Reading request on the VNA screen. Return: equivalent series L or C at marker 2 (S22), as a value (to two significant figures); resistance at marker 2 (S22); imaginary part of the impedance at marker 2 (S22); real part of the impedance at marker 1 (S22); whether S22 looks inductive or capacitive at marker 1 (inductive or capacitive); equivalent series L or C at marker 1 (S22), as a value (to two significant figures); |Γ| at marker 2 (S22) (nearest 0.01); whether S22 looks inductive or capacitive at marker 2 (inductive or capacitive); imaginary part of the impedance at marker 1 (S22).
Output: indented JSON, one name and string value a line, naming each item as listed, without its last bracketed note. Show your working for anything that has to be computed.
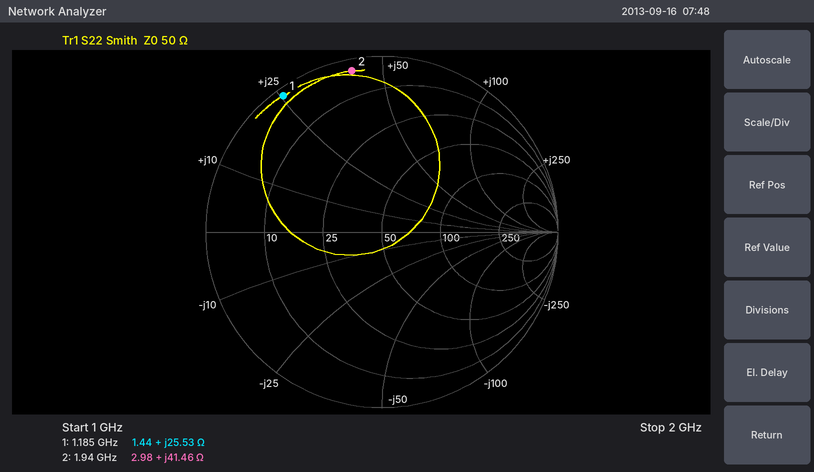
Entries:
{
  "equivalent series L or C at marker 2 (S22), as a value": "L = 41.46 Ω/(2π × 1.94 GHz) ≈ 3.4 nH",
  "resistance at marker 2": "2.98 Ω",
  "imaginary part of the impedance at marker 2": "+41.46 Ω",
  "real part of the impedance at marker 1": "1.44 Ω",
  "whether S22 looks inductive or capacitive at marker 1": "inductive",
  "equivalent series L or C at marker 1 (S22), as a value": "L = 25.53 Ω/(2π × 1.185 GHz) ≈ 3.4 nH",
  "|Γ| at marker 2 (S22)": "0.93",
  "whether S22 looks inductive or capacitive at marker 2": "inductive",
  "imaginary part of the impedance at marker 1": "+25.53 Ω"
}
